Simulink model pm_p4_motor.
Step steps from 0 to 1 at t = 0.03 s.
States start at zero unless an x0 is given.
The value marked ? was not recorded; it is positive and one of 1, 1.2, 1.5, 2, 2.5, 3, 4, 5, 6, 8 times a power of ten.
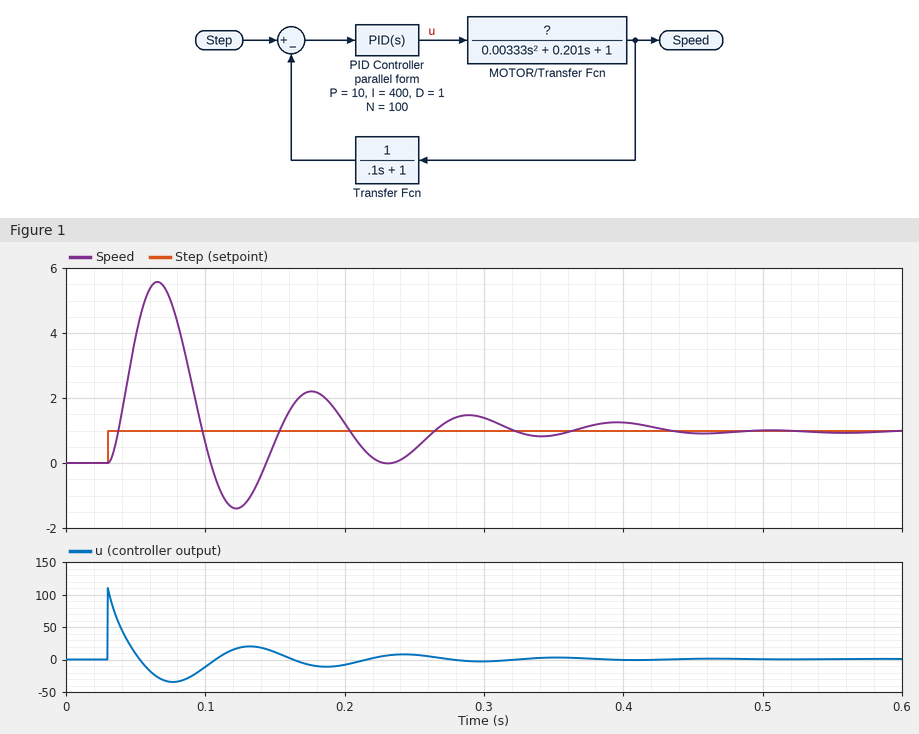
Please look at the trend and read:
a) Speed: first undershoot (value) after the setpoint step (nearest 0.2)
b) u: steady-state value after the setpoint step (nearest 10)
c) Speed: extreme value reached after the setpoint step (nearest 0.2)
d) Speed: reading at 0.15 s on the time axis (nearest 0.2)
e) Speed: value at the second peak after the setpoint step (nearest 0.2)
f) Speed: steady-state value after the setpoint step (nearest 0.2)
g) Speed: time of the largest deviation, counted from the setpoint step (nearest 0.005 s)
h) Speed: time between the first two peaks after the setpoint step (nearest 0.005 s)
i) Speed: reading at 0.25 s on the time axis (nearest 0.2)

-1.4
0
5.6
0.6
2.2
1.0
0.035 s
0.110 s
0.4
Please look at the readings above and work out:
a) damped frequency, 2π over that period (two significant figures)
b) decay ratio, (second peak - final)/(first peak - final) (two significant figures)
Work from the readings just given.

57 rad/s
0.26
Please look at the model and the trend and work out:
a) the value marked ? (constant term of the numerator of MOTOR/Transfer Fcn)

1.5
